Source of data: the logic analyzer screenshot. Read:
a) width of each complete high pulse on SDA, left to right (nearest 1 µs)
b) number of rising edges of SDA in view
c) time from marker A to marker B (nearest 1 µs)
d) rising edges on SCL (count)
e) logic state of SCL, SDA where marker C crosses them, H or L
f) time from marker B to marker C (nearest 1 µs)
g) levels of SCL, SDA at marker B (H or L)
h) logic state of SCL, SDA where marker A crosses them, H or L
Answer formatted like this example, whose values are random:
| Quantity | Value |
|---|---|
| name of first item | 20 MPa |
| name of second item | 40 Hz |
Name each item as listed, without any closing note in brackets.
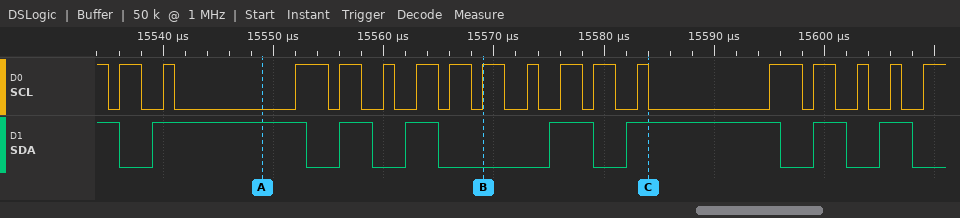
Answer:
| Quantity | Value |
|---|---|
| width of each complete high pulse on SDA, left to right | 14 µs, 3 µs, 3 µs, 4 µs, 14 µs, 3 µs, 3 µs |
| number of rising edges of SDA in view | 7 |
| time from marker A to marker B | 20 µs |
| rising edges on SCL | 17 |
| logic state of SCL, SDA where marker C crosses them, H or L | SCL=L, SDA=H |
| time from marker B to marker C | 15 µs |
| levels of SCL, SDA at marker B | SCL=H, SDA=L |
| logic state of SCL, SDA where marker A crosses them, H or L | SCL=L, SDA=H |
